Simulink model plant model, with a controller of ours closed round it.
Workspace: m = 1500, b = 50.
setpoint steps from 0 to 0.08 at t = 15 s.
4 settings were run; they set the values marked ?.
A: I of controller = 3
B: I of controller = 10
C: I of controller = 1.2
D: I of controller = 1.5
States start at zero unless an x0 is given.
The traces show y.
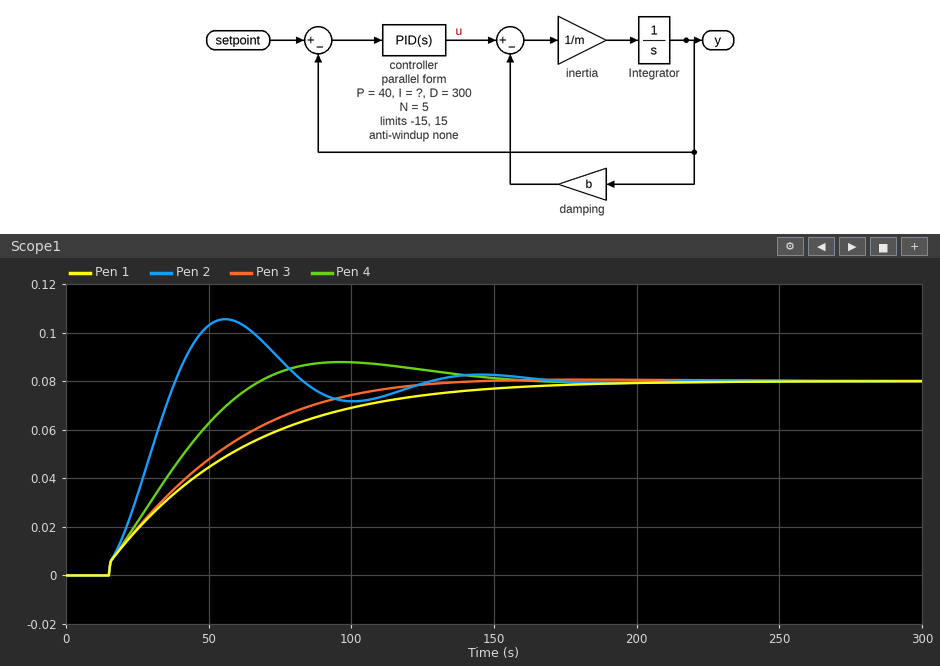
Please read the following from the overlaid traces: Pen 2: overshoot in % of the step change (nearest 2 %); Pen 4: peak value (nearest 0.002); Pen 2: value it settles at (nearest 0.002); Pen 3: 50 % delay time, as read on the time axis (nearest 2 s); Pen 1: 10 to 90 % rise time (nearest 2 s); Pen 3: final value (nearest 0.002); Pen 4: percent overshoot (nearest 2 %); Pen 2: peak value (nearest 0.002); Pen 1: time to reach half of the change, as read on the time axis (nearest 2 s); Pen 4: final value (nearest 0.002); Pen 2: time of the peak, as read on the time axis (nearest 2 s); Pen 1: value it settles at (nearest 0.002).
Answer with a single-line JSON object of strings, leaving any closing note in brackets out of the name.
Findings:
{"Pen 2: overshoot in % of the step change": "32 %", "Pen 4: peak value": "0.088", "Pen 2: value it settles at": "0.080", "Pen 3: 50 % delay time, as read on the time axis": "42 s", "Pen 1: 10 to 90 % rise time": "96 s", "Pen 3: final value": "0.080", "Pen 4: percent overshoot": "10 %", "Pen 2: peak value": "0.106", "Pen 1: time to reach half of the change, as read on the time axis": "44 s", "Pen 4: final value": "0.080", "Pen 2: time of the peak, as read on the time axis": "56 s", "Pen 1: value it settles at": "0.080"}
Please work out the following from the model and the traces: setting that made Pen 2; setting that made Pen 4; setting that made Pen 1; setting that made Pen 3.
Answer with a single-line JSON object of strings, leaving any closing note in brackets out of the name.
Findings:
{"setting that made Pen 2": "B", "setting that made Pen 4": "A", "setting that made Pen 1": "C", "setting that made Pen 3": "D"}
